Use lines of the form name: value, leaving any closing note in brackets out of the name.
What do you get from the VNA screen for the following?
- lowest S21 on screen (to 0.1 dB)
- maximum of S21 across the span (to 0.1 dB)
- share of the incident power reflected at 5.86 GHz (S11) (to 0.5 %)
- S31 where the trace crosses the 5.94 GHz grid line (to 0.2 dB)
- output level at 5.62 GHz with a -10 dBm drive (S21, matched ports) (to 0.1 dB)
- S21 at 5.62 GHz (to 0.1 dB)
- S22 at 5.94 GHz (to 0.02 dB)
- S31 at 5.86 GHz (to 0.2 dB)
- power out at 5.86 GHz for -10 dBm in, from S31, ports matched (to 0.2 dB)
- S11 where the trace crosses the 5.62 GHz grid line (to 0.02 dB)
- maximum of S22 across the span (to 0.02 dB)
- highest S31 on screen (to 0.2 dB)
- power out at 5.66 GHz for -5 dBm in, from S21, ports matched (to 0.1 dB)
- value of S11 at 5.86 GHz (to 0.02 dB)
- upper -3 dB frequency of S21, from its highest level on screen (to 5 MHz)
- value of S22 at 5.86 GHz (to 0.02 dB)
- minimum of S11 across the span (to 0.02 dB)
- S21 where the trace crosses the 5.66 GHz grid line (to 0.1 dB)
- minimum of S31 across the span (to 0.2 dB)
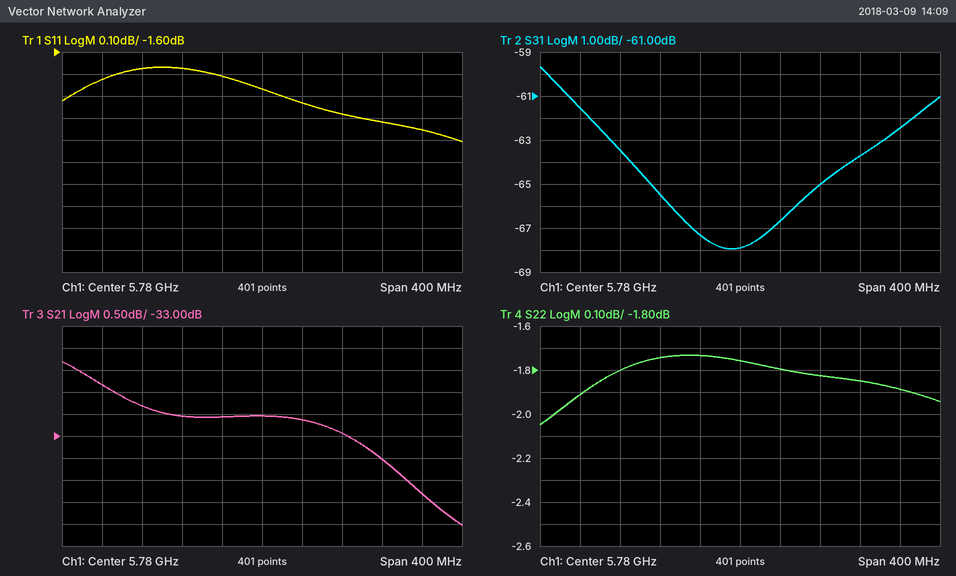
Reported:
lowest S21 on screen: -35.0 dB
maximum of S21 across the span: -31.3 dB
share of the incident power reflected at 5.86 GHz (S11): 65.0 %
S31 where the trace crosses the 5.94 GHz grid line: -62.4 dB
output level at 5.62 GHz with a -10 dBm drive (S21, matched ports): -41.8 dBm
S21 at 5.62 GHz: -31.8 dB
S22 at 5.94 GHz: -1.88 dB
S31 at 5.86 GHz: -65.0 dB
power out at 5.86 GHz for -10 dBm in, from S31, ports matched: -75.0 dBm
S11 where the trace crosses the 5.62 GHz grid line: -1.72 dB
maximum of S22 across the span: -1.74 dB
highest S31 on screen: -59.6 dB
power out at 5.66 GHz for -5 dBm in, from S21, ports matched: -37.3 dBm
value of S11 at 5.86 GHz: -1.88 dB
upper -3 dB frequency of S21, from its highest level on screen: 5.940 GHz
value of S22 at 5.86 GHz: -1.82 dB
minimum of S11 across the span: -2.00 dB
S21 where the trace crosses the 5.66 GHz grid line: -32.3 dB
minimum of S31 across the span: -68.0 dB
